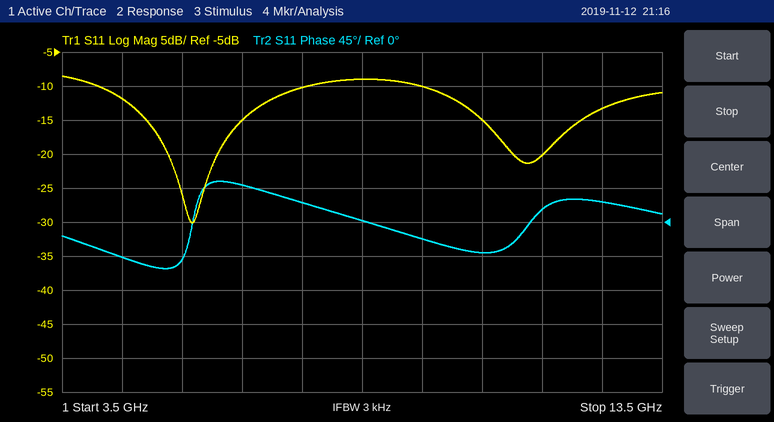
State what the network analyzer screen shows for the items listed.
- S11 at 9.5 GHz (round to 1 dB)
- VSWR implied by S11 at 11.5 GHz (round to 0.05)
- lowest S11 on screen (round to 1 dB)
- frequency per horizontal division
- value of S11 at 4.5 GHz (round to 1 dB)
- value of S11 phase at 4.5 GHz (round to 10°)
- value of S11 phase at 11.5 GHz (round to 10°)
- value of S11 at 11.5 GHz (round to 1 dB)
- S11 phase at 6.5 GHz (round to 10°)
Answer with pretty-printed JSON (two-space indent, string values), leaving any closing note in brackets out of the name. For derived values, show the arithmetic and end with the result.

{
  "S11 at 9.5 GHz": "-10 dB",
  "VSWR implied by S11 at 11.5 GHz": "|Γ| = 10^(-20/20) = 0.1000; VSWR = (1 + 0.1000)/(1 − 0.1000) ≈ 1.22, so 1.20 to the nearest 0.05",
  "lowest S11 on screen": "-30 dB",
  "frequency per horizontal division": "1 GHz",
  "value of S11 at 4.5 GHz": "-12 dB",
  "value of S11 phase at 4.5 GHz": "-50°",
  "value of S11 phase at 11.5 GHz": "20°",
  "value of S11 at 11.5 GHz": "-20 dB",
  "S11 phase at 6.5 GHz": "50°"
}
